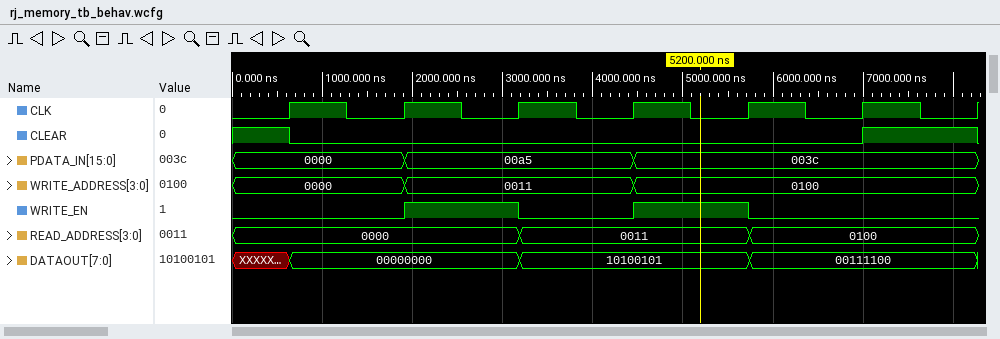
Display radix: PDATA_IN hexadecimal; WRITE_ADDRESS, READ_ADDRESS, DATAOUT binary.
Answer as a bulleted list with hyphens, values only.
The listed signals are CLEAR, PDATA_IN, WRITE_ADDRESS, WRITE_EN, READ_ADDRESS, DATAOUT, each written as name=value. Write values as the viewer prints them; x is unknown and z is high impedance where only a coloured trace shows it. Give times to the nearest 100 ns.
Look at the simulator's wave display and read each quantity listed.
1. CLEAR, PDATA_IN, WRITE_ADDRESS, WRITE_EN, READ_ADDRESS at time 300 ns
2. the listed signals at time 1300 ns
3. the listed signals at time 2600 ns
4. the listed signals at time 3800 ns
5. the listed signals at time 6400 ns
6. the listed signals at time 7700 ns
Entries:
- CLEAR=1, PDATA_IN=0000, WRITE_ADDRESS=0000, WRITE_EN=0, READ_ADDRESS=0000
- CLEAR=0, PDATA_IN=0000, WRITE_ADDRESS=0000, WRITE_EN=0, READ_ADDRESS=0000, DATAOUT=00000000
- CLEAR=0, PDATA_IN=00a5, WRITE_ADDRESS=0011, WRITE_EN=1, READ_ADDRESS=0000, DATAOUT=00000000
- CLEAR=0, PDATA_IN=00a5, WRITE_ADDRESS=0011, WRITE_EN=0, READ_ADDRESS=0011, DATAOUT=10100101
- CLEAR=0, PDATA_IN=003c, WRITE_ADDRESS=0100, WRITE_EN=0, READ_ADDRESS=0100, DATAOUT=00111100
- CLEAR=1, PDATA_IN=003c, WRITE_ADDRESS=0100, WRITE_EN=0, READ_ADDRESS=0100, DATAOUT=00111100
